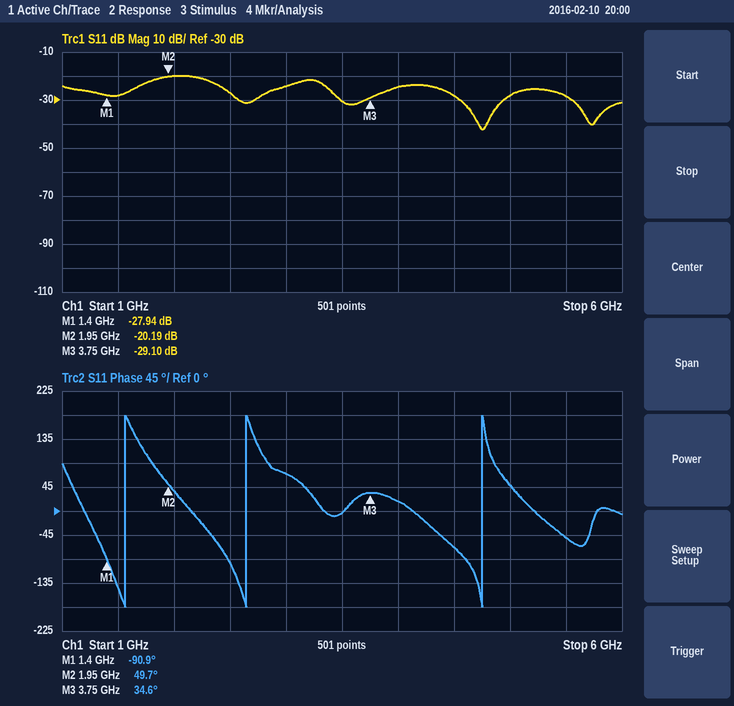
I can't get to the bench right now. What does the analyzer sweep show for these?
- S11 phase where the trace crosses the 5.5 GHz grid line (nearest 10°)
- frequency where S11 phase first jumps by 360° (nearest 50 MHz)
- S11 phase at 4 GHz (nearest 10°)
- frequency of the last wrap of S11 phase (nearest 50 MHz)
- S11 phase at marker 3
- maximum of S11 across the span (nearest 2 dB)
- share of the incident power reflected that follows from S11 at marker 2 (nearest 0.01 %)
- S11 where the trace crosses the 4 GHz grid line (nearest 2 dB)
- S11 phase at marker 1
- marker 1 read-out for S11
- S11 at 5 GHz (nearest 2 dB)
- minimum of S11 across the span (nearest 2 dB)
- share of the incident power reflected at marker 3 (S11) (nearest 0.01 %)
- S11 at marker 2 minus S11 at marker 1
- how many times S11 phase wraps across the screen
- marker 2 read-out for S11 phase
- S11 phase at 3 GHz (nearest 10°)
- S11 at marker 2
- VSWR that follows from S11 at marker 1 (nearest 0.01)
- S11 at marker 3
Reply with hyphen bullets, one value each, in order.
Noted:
- -50°
- 1.55 GHz
- 20°
- 4.75 GHz
- 34.6°
- -20 dB
- 0.96 %
- -24 dB
- -90.9°
- -27.94 dB
- -28 dB
- -42 dB
- 0.12 %
- 7.75 dB
- 3
- 49.7°
- 70°
- -20.19 dB
- 1.08
- -29.10 dB
